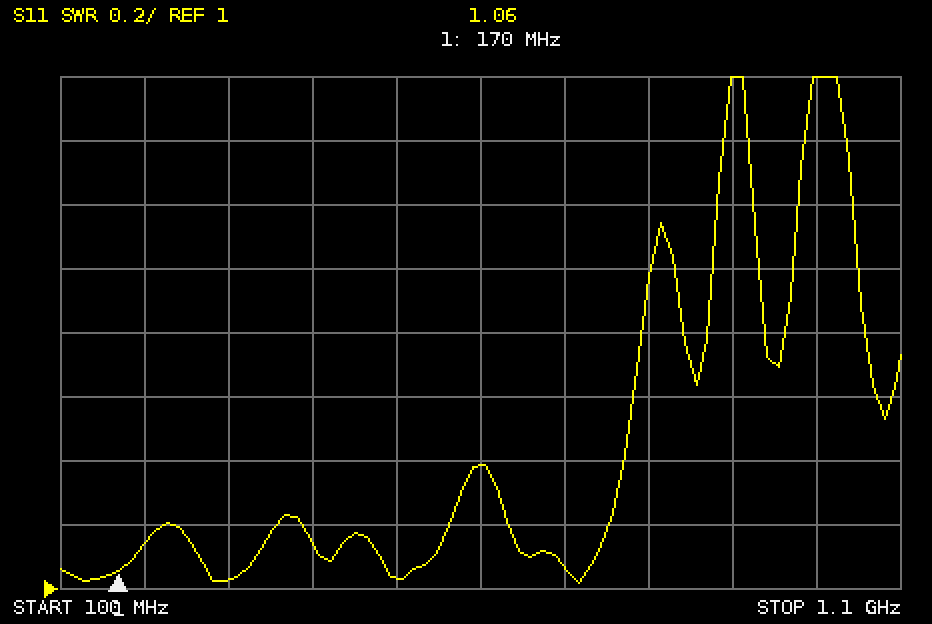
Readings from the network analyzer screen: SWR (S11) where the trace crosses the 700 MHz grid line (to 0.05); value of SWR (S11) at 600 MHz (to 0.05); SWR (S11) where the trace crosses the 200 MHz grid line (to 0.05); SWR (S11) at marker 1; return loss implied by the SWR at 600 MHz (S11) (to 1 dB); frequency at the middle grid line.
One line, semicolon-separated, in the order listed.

1.05; 1.40; 1.15; 1.06; 16 dB; 600 MHz
